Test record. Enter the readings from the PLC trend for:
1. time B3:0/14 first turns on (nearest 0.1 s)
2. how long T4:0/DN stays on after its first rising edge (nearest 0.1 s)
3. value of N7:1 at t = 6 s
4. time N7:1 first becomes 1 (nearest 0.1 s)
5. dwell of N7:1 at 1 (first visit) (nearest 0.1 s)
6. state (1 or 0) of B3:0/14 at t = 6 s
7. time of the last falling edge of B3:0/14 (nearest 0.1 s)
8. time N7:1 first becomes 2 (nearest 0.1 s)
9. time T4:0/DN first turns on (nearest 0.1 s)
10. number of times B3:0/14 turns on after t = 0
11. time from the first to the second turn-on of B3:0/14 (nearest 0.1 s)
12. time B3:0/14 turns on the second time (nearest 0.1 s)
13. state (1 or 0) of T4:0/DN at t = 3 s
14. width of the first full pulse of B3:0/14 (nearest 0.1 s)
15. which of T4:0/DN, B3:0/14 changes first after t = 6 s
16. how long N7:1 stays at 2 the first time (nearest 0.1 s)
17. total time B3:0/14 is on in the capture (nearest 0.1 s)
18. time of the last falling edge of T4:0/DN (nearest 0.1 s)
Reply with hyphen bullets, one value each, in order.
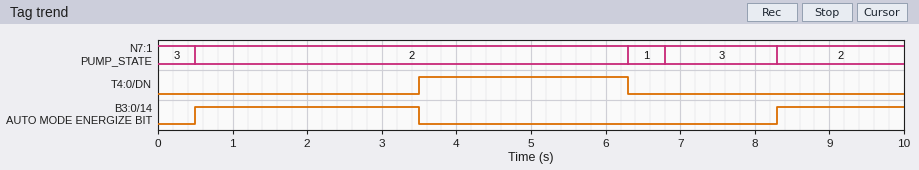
- 0.5 s
- 2.8 s
- 2
- 6.3 s
- 0.5 s
- 0
- 3.5 s
- 0.5 s
- 3.5 s
- 2
- 7.8 s
- 8.3 s
- 0
- 3.0 s
- T4:0/DN
- 5.8 s
- 4.7 s
- 6.3 s
